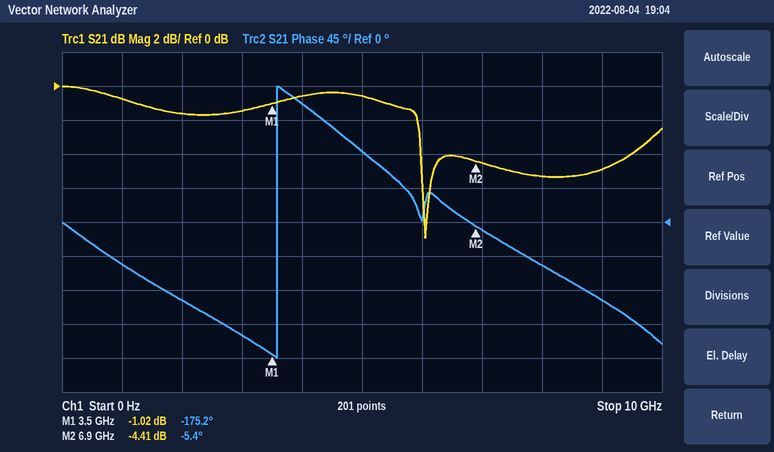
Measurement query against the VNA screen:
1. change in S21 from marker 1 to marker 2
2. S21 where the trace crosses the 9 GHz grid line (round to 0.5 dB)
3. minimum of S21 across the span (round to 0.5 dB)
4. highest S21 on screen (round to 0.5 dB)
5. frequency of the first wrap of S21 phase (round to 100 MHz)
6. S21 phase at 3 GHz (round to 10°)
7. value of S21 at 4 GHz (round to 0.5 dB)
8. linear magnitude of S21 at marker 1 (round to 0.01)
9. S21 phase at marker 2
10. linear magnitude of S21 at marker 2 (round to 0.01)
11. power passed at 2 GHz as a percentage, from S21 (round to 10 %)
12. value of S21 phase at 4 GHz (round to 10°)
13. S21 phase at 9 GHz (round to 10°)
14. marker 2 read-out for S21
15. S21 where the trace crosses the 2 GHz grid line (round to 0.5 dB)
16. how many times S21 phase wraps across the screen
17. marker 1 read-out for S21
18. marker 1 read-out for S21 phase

-3.39 dB
-5.0 dB
-9.0 dB
0.0 dB
3.6 GHz
-150°
-0.5 dB
0.89
-5.4°
0.60
70 %
160°
-100°
-4.41 dB
-1.5 dB
1
-1.02 dB
-175.2°
